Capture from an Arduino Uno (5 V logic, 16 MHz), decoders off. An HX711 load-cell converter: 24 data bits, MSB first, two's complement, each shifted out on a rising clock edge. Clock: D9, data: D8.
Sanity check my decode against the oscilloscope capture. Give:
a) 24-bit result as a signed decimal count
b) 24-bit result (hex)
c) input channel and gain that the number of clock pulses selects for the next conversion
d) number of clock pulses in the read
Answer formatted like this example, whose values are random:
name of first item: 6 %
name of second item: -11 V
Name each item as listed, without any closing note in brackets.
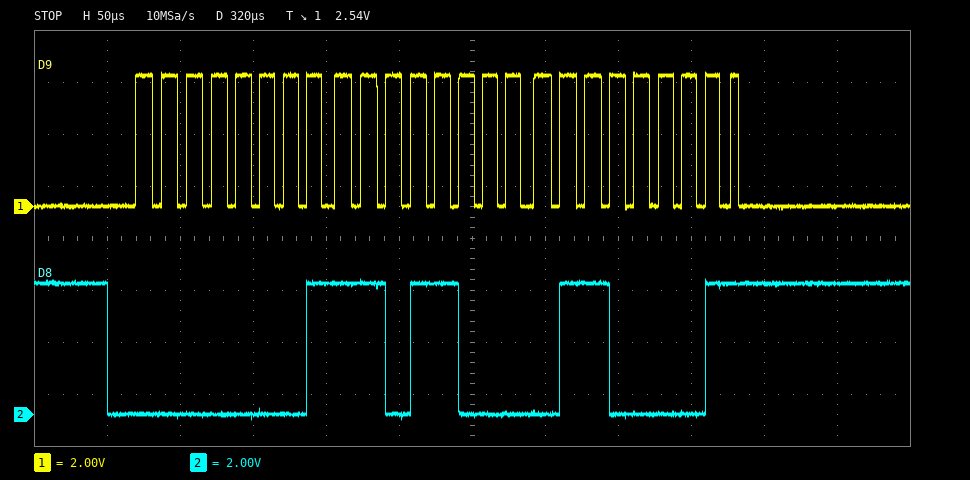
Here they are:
24-bit result as a signed decimal count: 120929
24-bit result: 0x01D861
input channel and gain that the number of clock pulses selects for the next conversion: channel A, gain 128
number of clock pulses in the read: 25
